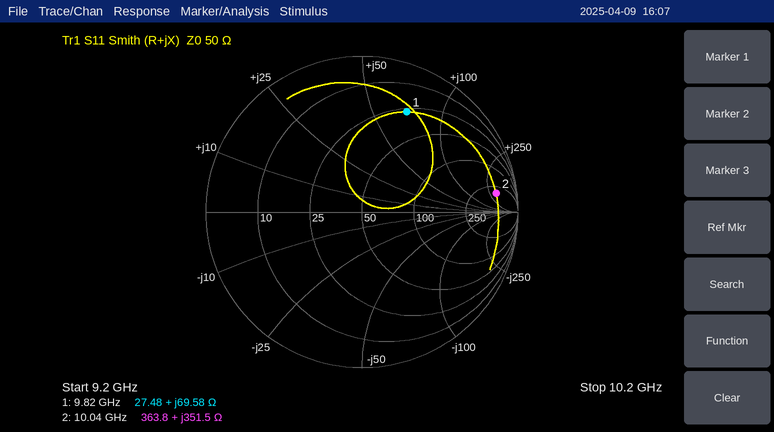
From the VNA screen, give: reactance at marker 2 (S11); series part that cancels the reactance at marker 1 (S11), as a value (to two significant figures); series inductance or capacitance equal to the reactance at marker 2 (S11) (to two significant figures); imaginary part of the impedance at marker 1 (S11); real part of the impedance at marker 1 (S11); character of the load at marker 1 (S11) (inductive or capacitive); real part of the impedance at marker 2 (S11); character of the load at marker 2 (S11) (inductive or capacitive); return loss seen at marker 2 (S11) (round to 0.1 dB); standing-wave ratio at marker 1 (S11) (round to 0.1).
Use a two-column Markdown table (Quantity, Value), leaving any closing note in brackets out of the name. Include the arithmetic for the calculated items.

| Quantity | Value |
|---|---|
| reactance at marker 2 | +351.5 Ω |
| series part that cancels the reactance at marker 1 (S11), as a value | C = 1/(2π × 9.82 GHz × 69.58 Ω) ≈ 233 fF, so 230 fF to two significant figures |
| series inductance or capacitance equal to the reactance at marker 2 (S11) | L = 351.5 Ω/(2π × 10.04 GHz) ≈ 5.6 nH |
| imaginary part of the impedance at marker 1 | +69.58 Ω |
| real part of the impedance at marker 1 | 27.48 Ω |
| character of the load at marker 1 (S11) | inductive |
| real part of the impedance at marker 2 | 363.8 Ω |
| character of the load at marker 2 (S11) | inductive |
| return loss seen at marker 2 (S11) | 1.2 dB |
| standing-wave ratio at marker 1 (S11) | 5.7 |
